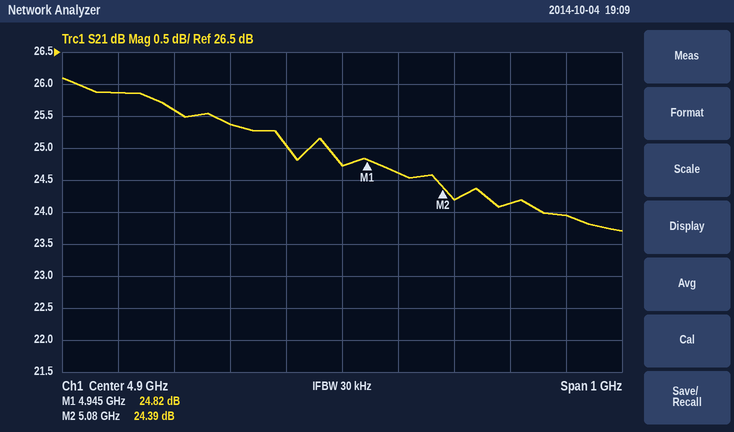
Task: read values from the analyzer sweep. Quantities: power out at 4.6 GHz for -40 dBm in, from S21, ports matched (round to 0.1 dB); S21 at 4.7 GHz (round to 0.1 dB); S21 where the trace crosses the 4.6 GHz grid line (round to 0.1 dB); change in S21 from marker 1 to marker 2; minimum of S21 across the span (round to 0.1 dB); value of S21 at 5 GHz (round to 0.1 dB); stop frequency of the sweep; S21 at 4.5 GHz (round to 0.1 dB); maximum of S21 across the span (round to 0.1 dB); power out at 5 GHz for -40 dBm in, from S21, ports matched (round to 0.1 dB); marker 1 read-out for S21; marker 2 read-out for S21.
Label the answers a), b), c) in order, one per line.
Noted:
a) -14.4 dBm
b) 25.4 dB
c) 25.6 dB
d) -0.43 dB
e) 23.7 dB
f) 24.6 dB
g) 5.4 GHz
h) 25.9 dB
i) 26.1 dB
j) -15.4 dBm
k) 24.82 dB
l) 24.39 dB
